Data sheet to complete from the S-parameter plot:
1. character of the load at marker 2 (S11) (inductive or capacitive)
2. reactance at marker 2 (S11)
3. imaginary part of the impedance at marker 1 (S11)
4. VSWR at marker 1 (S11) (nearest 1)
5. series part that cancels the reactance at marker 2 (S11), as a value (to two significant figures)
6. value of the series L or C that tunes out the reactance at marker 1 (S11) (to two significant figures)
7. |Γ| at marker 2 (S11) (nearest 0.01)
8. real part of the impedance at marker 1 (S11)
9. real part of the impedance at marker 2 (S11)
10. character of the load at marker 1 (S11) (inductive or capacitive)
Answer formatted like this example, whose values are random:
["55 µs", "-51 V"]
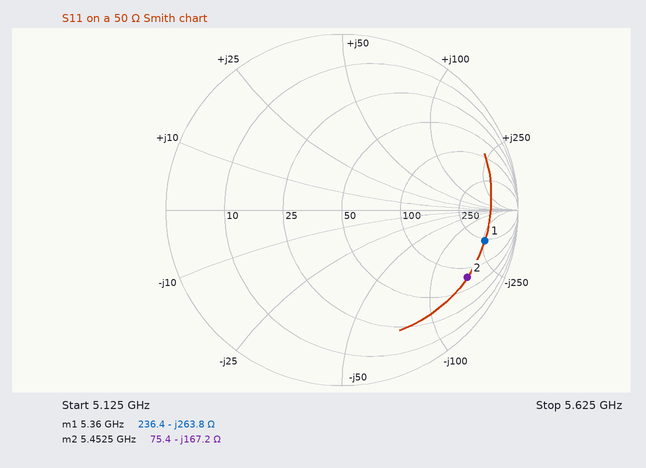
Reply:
["capacitive", "-167.2 Ω", "-263.8 Ω", "11", "4.9 nH", "7.8 nH", "0.81", "236.4 Ω", "75.4 Ω", "capacitive"]
